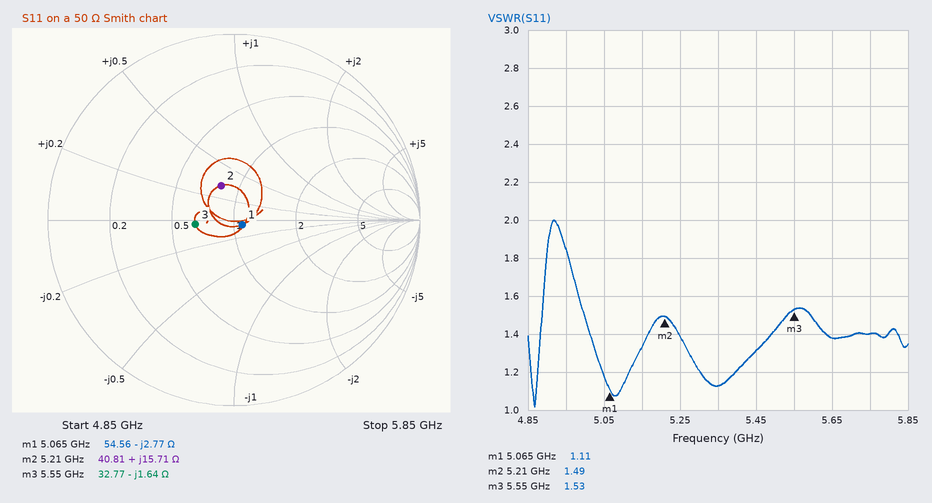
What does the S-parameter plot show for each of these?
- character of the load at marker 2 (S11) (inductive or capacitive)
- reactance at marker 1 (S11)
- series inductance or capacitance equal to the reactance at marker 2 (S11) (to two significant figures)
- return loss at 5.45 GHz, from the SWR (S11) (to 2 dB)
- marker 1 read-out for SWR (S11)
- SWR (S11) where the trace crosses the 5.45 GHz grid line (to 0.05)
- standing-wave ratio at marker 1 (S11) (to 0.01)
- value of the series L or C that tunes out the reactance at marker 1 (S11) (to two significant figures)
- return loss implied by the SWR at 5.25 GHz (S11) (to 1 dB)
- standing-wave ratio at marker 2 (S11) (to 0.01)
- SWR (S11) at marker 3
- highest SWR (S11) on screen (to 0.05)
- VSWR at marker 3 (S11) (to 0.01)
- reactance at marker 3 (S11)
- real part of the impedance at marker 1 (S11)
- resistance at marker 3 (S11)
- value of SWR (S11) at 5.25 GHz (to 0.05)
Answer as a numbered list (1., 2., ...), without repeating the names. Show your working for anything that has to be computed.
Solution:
1. inductive
2. -2.77 Ω
3. L = 15.71 Ω/(2π × 5.21 GHz) ≈ 480 pH
4. −20 log10((1.3 − 1)/(1.3 + 1)) ≈ 18 dB
5. 1.11
6. 1.30
7. 1.11
8. L = 2.77 Ω/(2π × 5.065 GHz) ≈ 87 pH
9. −20 log10((1.4 − 1)/(1.4 + 1)) ≈ 16 dB
10. 1.49
11. 1.53
12. 2.00
13. 1.53
14. -1.64 Ω
15. 54.56 Ω
16. 32.77 Ω
17. 1.40
